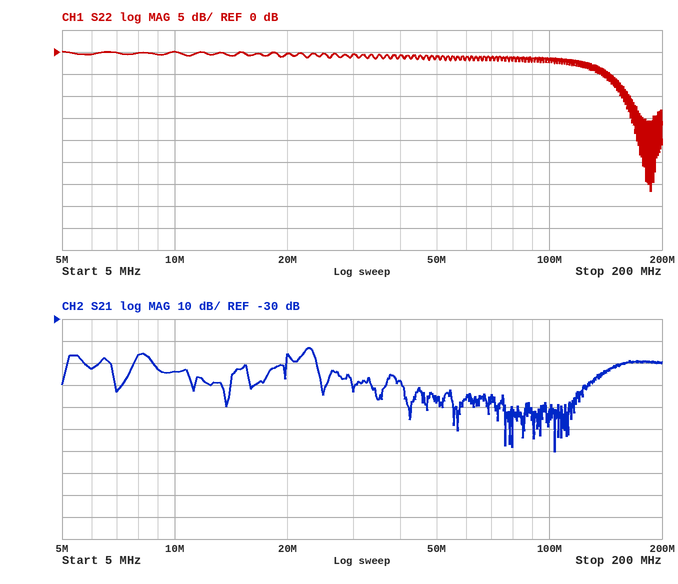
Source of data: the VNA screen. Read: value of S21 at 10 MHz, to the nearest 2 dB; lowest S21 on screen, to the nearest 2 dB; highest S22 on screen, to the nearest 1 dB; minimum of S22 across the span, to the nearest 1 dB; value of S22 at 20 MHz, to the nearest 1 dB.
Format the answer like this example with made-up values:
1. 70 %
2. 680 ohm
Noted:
1. -54 dB
2. -90 dB
3. 0 dB
4. -32 dB
5. 0 dB
